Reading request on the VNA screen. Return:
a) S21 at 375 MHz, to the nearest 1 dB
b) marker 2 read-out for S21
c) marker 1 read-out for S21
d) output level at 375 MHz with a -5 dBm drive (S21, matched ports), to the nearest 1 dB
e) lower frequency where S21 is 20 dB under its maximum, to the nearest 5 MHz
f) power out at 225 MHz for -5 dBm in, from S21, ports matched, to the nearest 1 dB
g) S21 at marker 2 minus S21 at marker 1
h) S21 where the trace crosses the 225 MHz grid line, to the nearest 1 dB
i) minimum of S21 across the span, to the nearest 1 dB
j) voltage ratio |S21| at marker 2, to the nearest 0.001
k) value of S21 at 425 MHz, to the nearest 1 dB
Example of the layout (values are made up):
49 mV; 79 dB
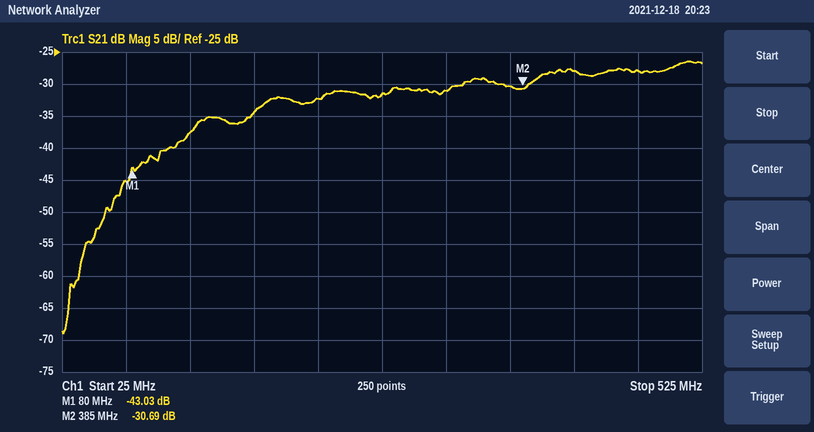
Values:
-30 dB; -30.69 dB; -43.03 dB; -35 dBm; 70 MHz; -37 dBm; 12.34 dB; -32 dB; -69 dB; 0.029; -28 dB
